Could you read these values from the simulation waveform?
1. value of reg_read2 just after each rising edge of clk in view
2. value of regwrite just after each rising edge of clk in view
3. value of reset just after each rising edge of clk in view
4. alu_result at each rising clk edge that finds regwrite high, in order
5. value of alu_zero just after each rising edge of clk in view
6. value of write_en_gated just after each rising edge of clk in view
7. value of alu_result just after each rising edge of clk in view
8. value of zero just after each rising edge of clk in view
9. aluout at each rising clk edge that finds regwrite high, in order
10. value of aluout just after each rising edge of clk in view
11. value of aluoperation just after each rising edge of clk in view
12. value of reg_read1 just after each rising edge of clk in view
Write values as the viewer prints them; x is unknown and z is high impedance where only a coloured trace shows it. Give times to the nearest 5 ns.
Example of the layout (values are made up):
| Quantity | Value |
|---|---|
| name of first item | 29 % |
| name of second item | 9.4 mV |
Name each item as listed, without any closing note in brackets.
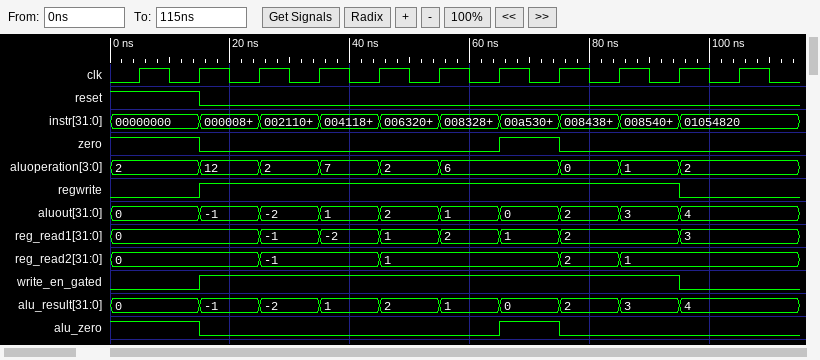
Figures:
| Quantity | Value |
|---|---|
| value of reg_read2 just after each rising edge of clk in view | 0, 0, -1, -1, 1, 1, 1, 2, 1, 1, 1 |
| value of regwrite just after each rising edge of clk in view | 0 1 1 1 1 1 1 1 1 0 0 |
| value of reset just after each rising edge of clk in view | 1 0 0 0 0 0 0 0 0 0 0 |
| alu_result at each rising clk edge that finds regwrite high, in order | -1, -2, 1, 2, 1, 0, 2, 3 |
| value of alu_zero just after each rising edge of clk in view | 1 0 0 0 0 0 1 0 0 0 0 |
| value of write_en_gated just after each rising edge of clk in view | 0 1 1 1 1 1 1 1 1 0 0 |
| value of alu_result just after each rising edge of clk in view | 0, -1, -2, 1, 2, 1, 0, 2, 3, 4, 4 |
| value of zero just after each rising edge of clk in view | 1 0 0 0 0 0 1 0 0 0 0 |
| aluout at each rising clk edge that finds regwrite high, in order | -1, -2, 1, 2, 1, 0, 2, 3 |
| value of aluout just after each rising edge of clk in view | 0, -1, -2, 1, 2, 1, 0, 2, 3, 4, 4 |
| value of aluoperation just after each rising edge of clk in view | 2, 12, 2, 7, 2, 6, 6, 0, 1, 2, 2 |
| value of reg_read1 just after each rising edge of clk in view | 0, 0, -1, -2, 1, 2, 1, 2, 2, 3, 3 |
